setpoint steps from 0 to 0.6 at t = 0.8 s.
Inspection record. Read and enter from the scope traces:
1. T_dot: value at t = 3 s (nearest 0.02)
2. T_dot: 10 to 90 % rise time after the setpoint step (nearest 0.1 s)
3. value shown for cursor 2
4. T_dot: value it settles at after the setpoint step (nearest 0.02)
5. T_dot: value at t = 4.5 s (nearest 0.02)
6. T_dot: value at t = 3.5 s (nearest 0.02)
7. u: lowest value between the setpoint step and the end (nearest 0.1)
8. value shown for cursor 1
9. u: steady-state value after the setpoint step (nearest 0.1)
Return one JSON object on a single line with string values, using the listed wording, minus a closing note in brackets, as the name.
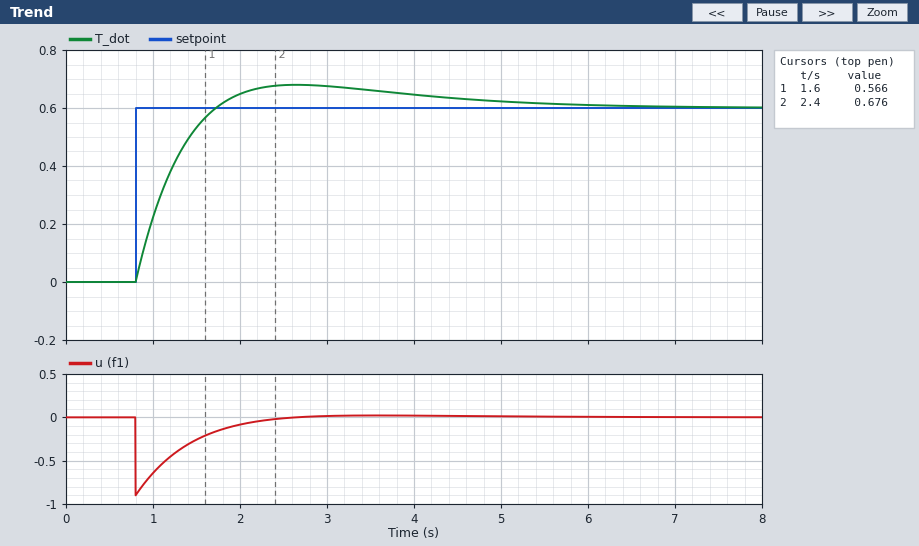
{"T_dot: value at t = 3 s": "0.68", "T_dot: 10 to 90 % rise time after the setpoint step": "0.7 s", "value shown for cursor 2": "0.676", "T_dot: value it settles at after the setpoint step": "0.60", "T_dot: value at t = 4.5 s": "0.64", "T_dot: value at t = 3.5 s": "0.66", "u: lowest value between the setpoint step and the end": "-0.9", "value shown for cursor 1": "0.566", "u: steady-state value after the setpoint step": "0.0"}
